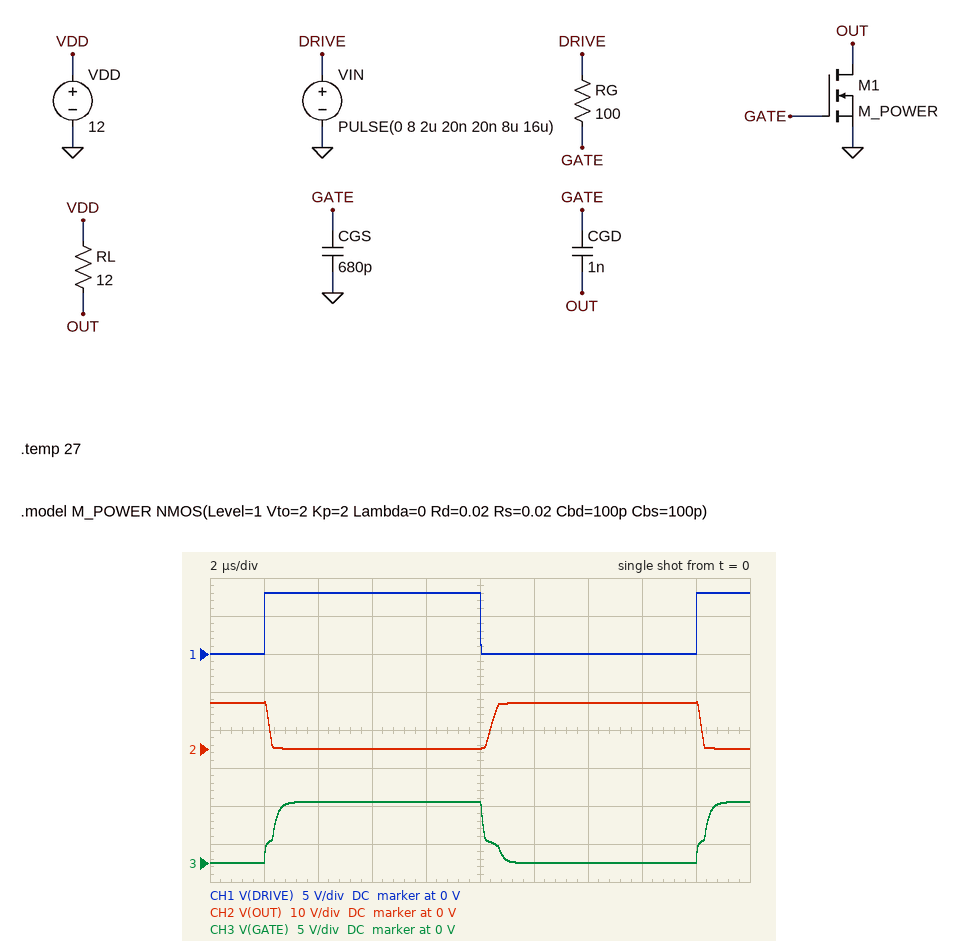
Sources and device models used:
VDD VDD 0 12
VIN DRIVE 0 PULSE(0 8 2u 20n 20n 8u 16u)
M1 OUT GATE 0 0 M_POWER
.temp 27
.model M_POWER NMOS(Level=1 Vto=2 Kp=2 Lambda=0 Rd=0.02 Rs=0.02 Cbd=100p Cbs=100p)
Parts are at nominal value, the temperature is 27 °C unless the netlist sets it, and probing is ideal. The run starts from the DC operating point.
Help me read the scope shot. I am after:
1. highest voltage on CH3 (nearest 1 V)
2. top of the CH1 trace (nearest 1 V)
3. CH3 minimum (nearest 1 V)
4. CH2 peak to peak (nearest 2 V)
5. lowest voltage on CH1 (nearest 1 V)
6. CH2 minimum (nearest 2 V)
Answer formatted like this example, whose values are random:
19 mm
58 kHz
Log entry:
8 V
8 V
0 V
12 V
0 V
0 V
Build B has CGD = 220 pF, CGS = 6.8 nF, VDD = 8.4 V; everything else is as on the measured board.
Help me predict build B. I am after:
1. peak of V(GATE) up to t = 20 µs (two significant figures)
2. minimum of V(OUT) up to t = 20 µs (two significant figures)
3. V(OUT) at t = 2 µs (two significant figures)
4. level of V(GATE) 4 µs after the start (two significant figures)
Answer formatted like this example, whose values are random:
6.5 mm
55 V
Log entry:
8.0 V
86 mV
8.4 V
7.5 V
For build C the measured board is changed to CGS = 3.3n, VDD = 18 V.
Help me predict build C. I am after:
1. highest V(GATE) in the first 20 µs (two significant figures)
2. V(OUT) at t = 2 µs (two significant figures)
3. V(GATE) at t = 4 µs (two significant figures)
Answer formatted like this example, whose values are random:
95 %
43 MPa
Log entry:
8.0 V
18 V
7.8 V
